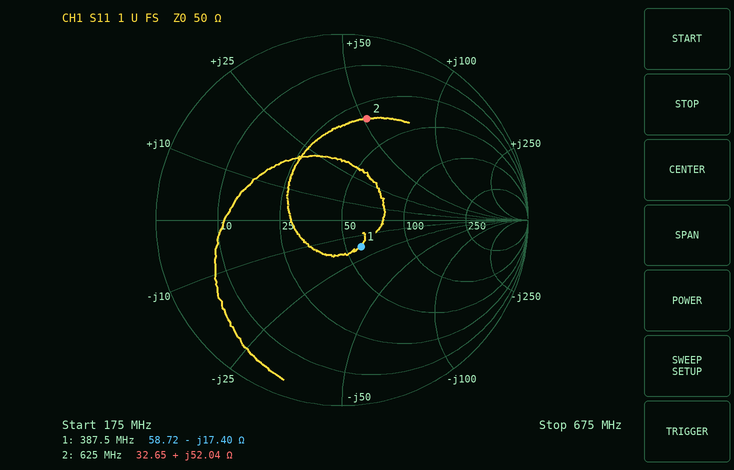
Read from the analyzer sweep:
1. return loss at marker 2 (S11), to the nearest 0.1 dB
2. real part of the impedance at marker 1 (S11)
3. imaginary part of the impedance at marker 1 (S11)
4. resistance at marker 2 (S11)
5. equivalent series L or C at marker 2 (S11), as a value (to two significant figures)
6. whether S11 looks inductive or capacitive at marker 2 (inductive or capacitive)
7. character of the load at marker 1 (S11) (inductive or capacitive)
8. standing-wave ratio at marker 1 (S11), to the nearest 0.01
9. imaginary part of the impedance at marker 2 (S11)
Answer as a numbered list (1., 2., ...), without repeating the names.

1. 5.0 dB
2. 58.72 Ω
3. -17.40 Ω
4. 32.65 Ω
5. 13 nH
6. inductive
7. capacitive
8. 1.43
9. +52.04 Ω
